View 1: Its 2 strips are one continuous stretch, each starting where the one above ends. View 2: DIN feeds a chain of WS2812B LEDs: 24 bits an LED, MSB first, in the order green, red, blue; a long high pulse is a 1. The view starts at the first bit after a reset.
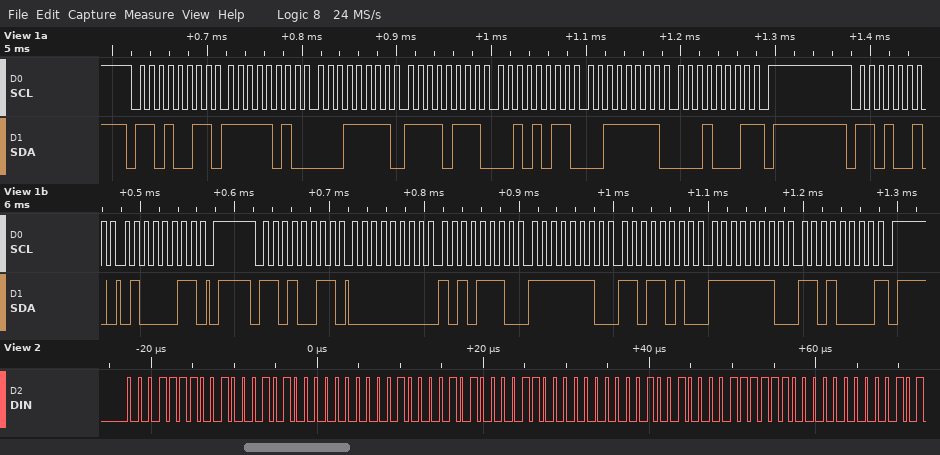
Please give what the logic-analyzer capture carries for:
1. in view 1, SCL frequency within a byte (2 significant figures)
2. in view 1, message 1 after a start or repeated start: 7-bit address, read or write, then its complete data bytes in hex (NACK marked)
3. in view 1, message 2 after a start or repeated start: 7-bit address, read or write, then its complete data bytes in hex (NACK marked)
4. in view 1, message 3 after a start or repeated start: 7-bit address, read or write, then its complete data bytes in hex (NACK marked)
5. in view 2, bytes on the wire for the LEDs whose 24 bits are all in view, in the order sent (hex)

100 kHz
0x69 read: FA 1F F7 2B 3F 11 NACK
0x69 write: 43
0x69 read: 00 AE FE DA FE D0 NACK
1E 45 00 21 43 00 24 3F 00
